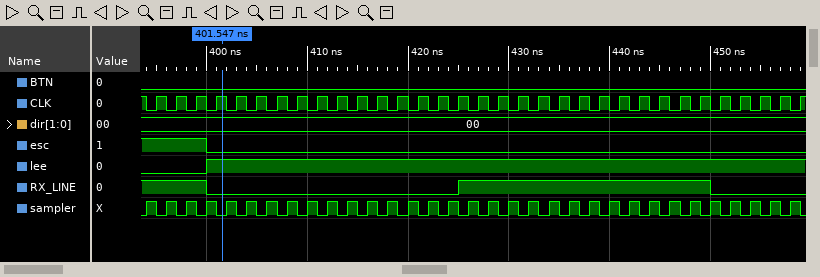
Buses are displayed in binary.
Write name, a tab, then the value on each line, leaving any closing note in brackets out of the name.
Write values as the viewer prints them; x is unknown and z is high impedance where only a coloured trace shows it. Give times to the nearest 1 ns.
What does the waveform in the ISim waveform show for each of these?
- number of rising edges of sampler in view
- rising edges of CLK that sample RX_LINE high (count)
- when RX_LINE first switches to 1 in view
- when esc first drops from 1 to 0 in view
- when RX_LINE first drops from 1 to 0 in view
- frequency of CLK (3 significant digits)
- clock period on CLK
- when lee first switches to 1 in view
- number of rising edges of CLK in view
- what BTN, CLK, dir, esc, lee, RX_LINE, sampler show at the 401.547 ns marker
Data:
number of rising edges of sampler in view	33
rising edges of CLK that sample RX_LINE high	15
when RX_LINE first switches to 1 in view	425 ns
when esc first drops from 1 to 0 in view	400 ns
when RX_LINE first drops from 1 to 0 in view	400 ns
frequency of CLK	500 MHz
clock period on CLK	2 ns
when lee first switches to 1 in view	400 ns
number of rising edges of CLK in view	33
what BTN, CLK, dir, esc, lee, RX_LINE, sampler show at the 401.547 ns marker	BTN=0, CLK=1, dir=00, esc=0, lee=1, RX_LINE=0, sampler=0
